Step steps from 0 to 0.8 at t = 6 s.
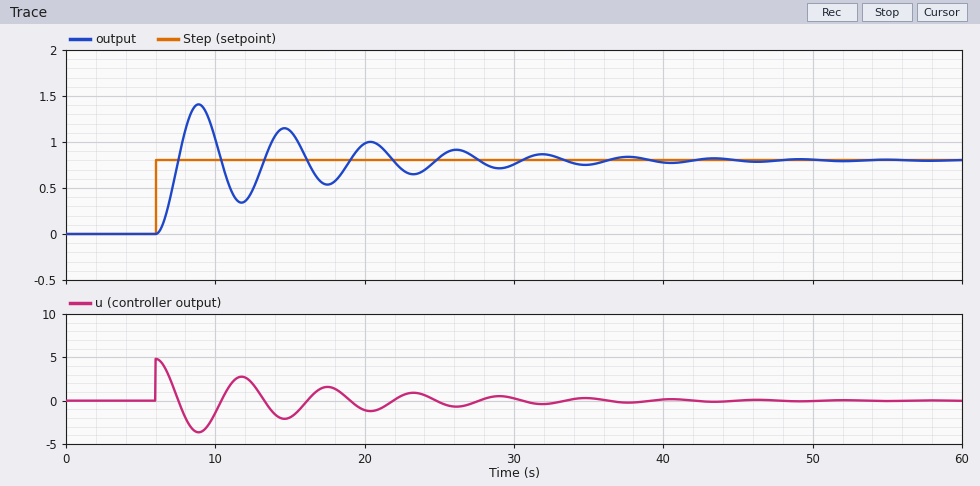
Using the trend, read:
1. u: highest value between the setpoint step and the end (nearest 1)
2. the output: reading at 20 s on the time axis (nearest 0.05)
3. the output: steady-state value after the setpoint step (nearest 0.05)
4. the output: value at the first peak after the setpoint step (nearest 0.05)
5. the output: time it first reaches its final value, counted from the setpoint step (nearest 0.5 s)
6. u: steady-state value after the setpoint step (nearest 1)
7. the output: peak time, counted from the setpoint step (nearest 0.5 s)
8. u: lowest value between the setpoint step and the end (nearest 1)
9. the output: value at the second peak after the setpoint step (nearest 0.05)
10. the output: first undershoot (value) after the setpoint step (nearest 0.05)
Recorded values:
5
1.00
0.80
1.40
1.5 s
0
3.0 s
-4
1.15
0.35
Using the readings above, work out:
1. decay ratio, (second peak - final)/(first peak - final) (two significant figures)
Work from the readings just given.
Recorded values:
0.58
